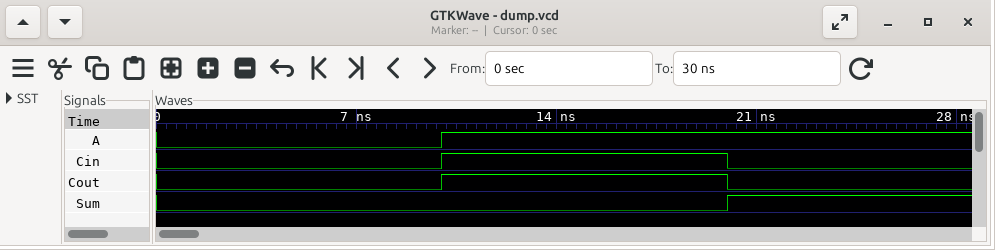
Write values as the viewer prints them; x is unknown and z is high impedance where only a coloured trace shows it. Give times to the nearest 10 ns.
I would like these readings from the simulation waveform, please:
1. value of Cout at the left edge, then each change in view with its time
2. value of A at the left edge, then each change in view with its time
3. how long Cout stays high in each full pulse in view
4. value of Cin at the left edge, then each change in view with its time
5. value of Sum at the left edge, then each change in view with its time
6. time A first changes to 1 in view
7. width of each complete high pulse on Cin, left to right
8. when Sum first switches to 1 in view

0, 1 at 10 ns, 0 at 20 ns
0, 1 at 10 ns
10 ns
0, 1 at 10 ns, 0 at 20 ns
0, 1 at 20 ns
10 ns
10 ns
20 ns
